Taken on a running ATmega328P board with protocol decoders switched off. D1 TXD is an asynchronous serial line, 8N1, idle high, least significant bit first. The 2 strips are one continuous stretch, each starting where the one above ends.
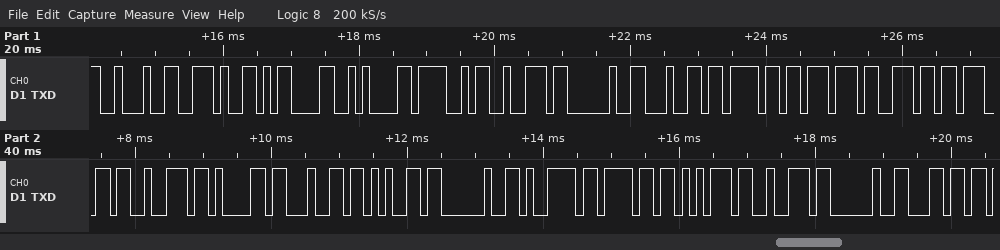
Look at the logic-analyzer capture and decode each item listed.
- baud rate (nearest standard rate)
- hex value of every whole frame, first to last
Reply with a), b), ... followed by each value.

a) 9600 baud
b) 22 2E 0D 0A 4F 72 20 64 6F 77 6E 67 72 61 64 65 20 79 6F 75 72 20 6C
